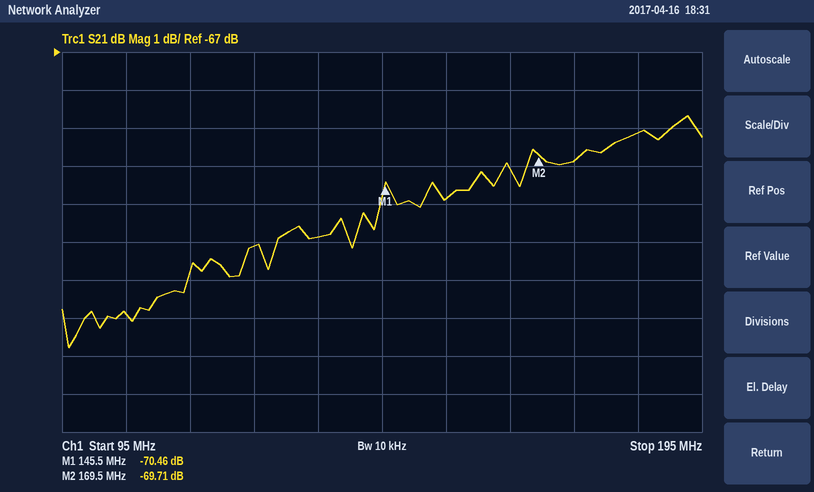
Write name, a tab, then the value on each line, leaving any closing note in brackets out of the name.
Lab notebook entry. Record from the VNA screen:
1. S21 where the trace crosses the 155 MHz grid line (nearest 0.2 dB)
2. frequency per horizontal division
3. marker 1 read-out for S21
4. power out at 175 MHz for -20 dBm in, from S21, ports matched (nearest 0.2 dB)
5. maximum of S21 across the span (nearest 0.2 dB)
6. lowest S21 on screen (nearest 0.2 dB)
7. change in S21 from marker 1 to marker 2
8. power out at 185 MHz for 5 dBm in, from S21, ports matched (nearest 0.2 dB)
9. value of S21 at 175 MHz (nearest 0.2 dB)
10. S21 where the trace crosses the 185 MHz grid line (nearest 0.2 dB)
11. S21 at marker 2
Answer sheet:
S21 where the trace crosses the 155 MHz grid line	-70.8 dB
frequency per horizontal division	10 MHz
marker 1 read-out for S21	-70.46 dB
power out at 175 MHz for -20 dBm in, from S21, ports matched	-89.8 dBm
maximum of S21 across the span	-68.6 dB
lowest S21 on screen	-74.8 dB
change in S21 from marker 1 to marker 2	0.75 dB
power out at 185 MHz for 5 dBm in, from S21, ports matched	-64.2 dBm
value of S21 at 175 MHz	-69.8 dB
S21 where the trace crosses the 185 MHz grid line	-69.2 dB
S21 at marker 2	-69.71 dB
